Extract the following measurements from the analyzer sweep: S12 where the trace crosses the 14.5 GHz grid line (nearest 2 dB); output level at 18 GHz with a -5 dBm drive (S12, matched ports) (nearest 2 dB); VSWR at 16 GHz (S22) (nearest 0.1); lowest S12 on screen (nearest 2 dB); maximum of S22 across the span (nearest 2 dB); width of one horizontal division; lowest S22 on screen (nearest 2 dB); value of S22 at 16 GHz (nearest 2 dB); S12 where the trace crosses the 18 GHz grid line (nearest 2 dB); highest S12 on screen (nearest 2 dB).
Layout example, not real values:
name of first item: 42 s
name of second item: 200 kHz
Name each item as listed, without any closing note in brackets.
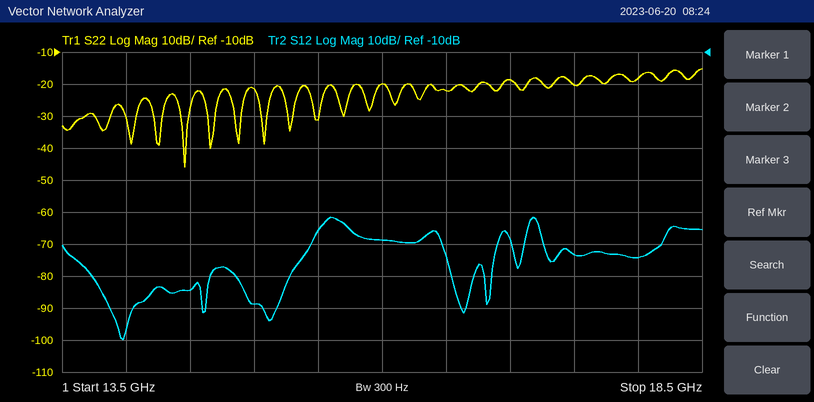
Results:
S12 where the trace crosses the 14.5 GHz grid line: -84 dB
output level at 18 GHz with a -5 dBm drive (S12, matched ports): -80 dBm
VSWR at 16 GHz (S22): 1.2
lowest S12 on screen: -100 dB
maximum of S22 across the span: -16 dB
width of one horizontal division: 500 MHz
lowest S22 on screen: -46 dB
value of S22 at 16 GHz: -20 dB
S12 where the trace crosses the 18 GHz grid line: -74 dB
highest S12 on screen: -62 dB
